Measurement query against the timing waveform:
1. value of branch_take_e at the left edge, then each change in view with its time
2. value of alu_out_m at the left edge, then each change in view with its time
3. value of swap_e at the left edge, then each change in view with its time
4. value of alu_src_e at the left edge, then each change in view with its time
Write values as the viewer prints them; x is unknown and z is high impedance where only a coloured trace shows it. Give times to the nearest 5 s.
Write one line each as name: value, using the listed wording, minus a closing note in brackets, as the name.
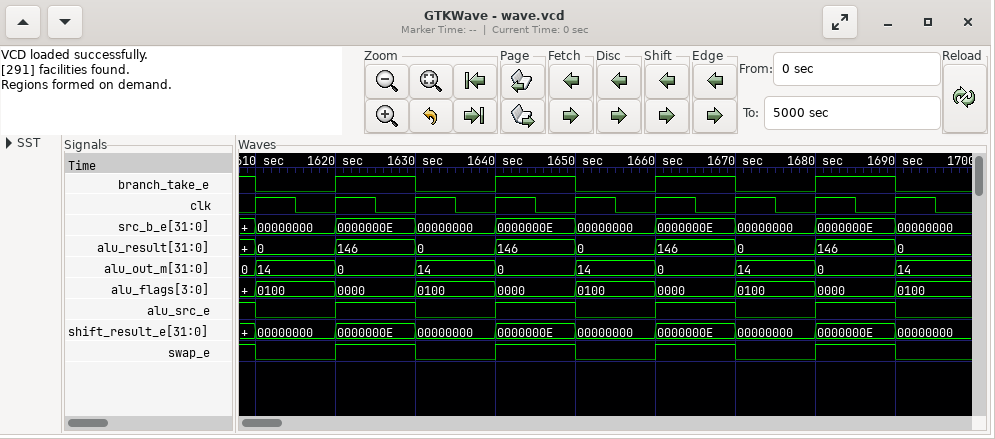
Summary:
value of branch_take_e at the left edge, then each change in view with its time: 1, 0 at 1610 s, 1 at 1620 s, 0 at 1630 s, 1 at 1640 s, 0 at 1650 s, 1 at 1660 s, 0 at 1670 s, 1 at 1680 s, 0 at 1690 s
value of alu_out_m at the left edge, then each change in view with its time: 0, 14 at 1610 s, 0 at 1620 s, 14 at 1630 s, 0 at 1640 s, 14 at 1650 s, 0 at 1660 s, 14 at 1670 s, 0 at 1680 s, 14 at 1690 s
value of swap_e at the left edge, then each change in view with its time: 1, 0 at 1610 s, 1 at 1620 s, 0 at 1630 s, 1 at 1640 s, 0 at 1650 s, 1 at 1660 s, 0 at 1670 s, 1 at 1680 s, 0 at 1690 s
value of alu_src_e at the left edge, then each change in view with its time: 1, 0 at 1610 s, 1 at 1620 s, 0 at 1630 s, 1 at 1640 s, 0 at 1650 s, 1 at 1660 s, 0 at 1670 s, 1 at 1680 s, 0 at 1690 s
